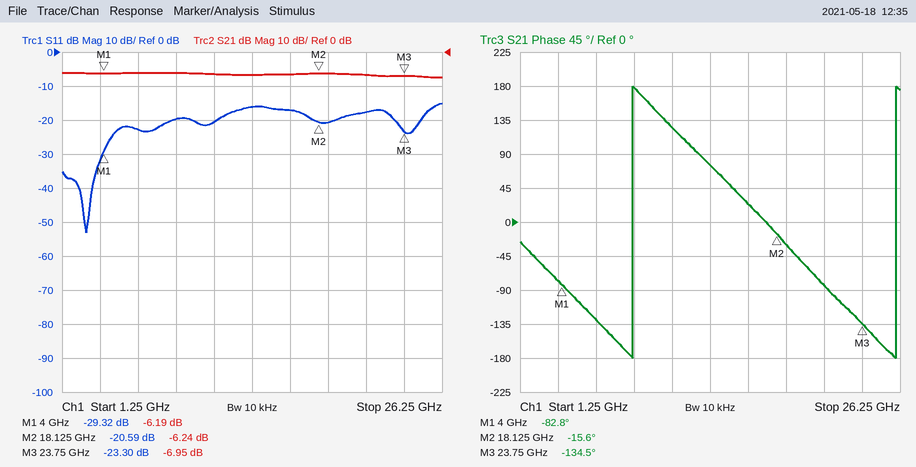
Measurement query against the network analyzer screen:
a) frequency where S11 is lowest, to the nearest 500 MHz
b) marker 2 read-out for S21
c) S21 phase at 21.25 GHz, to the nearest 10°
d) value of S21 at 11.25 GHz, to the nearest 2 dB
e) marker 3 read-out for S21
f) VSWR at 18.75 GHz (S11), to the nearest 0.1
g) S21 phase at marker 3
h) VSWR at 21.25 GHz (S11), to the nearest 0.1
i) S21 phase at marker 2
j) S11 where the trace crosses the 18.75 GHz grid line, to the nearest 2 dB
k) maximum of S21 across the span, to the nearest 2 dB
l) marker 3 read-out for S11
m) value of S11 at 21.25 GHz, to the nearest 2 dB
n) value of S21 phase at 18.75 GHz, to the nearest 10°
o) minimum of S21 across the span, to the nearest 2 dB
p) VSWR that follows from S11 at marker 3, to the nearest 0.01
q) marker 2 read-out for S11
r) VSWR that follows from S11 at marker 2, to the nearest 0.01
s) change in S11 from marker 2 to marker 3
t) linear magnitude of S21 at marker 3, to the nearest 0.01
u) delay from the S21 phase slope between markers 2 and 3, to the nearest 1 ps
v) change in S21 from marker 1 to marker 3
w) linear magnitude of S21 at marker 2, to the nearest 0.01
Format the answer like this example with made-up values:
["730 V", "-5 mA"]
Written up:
["3.0 GHz", "-6.24 dB", "-80°", "-6 dB", "-6.95 dB", "1.2", "-134.5°", "1.3", "-15.6°", "-20 dB", "-6 dB", "-23.30 dB", "-18 dB", "-30°", "-8 dB", "1.15", "-20.59 dB", "1.21", "-2.71 dB", "0.45", "59 ps", "-0.76 dB", "0.49"]
